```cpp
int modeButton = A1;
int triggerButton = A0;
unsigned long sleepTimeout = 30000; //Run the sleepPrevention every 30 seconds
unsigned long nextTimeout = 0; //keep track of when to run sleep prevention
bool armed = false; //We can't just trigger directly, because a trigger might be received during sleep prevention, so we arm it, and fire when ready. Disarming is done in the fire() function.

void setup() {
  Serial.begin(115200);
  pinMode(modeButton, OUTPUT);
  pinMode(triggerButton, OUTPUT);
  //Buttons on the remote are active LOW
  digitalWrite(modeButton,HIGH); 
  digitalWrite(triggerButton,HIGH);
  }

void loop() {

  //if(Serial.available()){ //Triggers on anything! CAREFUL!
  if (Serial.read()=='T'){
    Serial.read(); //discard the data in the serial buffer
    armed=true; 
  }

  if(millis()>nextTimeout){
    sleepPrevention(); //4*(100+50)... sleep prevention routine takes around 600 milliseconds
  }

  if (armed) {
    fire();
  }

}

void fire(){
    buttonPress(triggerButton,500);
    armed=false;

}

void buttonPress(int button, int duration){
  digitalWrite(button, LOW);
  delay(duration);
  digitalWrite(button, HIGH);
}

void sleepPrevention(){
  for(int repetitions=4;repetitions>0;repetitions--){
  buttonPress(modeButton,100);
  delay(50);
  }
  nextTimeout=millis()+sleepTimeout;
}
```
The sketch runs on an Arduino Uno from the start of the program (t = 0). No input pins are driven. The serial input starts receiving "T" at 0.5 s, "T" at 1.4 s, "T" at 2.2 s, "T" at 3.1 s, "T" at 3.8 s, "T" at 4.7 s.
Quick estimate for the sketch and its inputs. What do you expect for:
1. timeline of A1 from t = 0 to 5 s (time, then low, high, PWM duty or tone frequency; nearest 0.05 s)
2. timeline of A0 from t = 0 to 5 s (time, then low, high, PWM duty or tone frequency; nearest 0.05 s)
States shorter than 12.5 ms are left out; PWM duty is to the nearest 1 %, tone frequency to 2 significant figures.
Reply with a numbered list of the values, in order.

1. 0 s low; 0.1 s high; 0.15 s low; 0.25 s high; 0.3 s low; 0.4 s high; 0.45 s low; 0.55 s high
2. 0 s high; 0.6 s low; 1.1 s high; 1.4 s low; 1.9 s high; 2.2 s low; 2.7 s high; 3.1 s low; 3.6 s high; 3.8 s low; 4.3 s high; 4.7 s low
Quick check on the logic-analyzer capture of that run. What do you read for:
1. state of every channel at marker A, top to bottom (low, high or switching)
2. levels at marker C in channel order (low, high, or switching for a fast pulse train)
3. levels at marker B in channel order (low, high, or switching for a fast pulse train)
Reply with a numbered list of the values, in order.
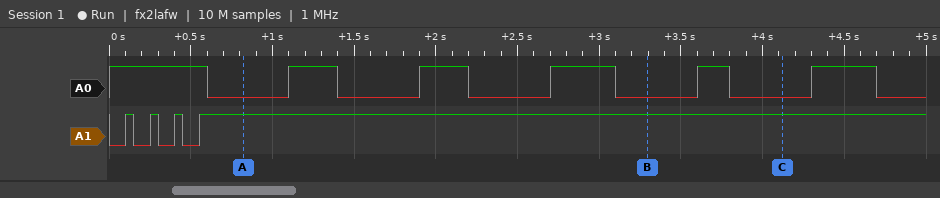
1. A0 low, A1 high
2. A0 low, A1 high
3. A0 low, A1 high
